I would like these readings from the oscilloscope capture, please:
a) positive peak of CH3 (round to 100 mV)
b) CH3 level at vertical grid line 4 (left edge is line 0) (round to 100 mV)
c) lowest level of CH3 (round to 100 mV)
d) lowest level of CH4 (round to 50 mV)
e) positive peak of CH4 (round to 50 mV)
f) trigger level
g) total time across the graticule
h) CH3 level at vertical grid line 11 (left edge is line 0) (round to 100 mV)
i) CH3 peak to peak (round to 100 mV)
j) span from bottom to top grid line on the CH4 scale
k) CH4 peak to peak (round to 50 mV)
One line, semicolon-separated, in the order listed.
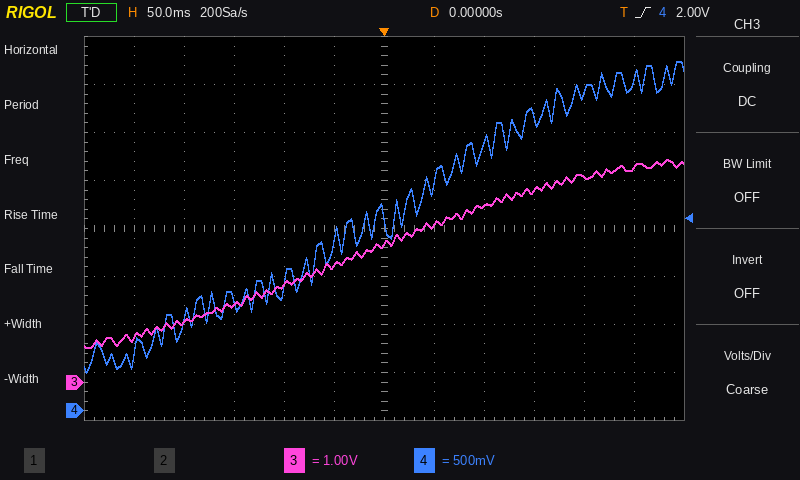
4.6 V; 2.0 V; 700 mV; 400 mV; 3.65 V; 2.00 V; 600 ms; 4.5 V; 3.9 V; 4 V; 3.25 V
